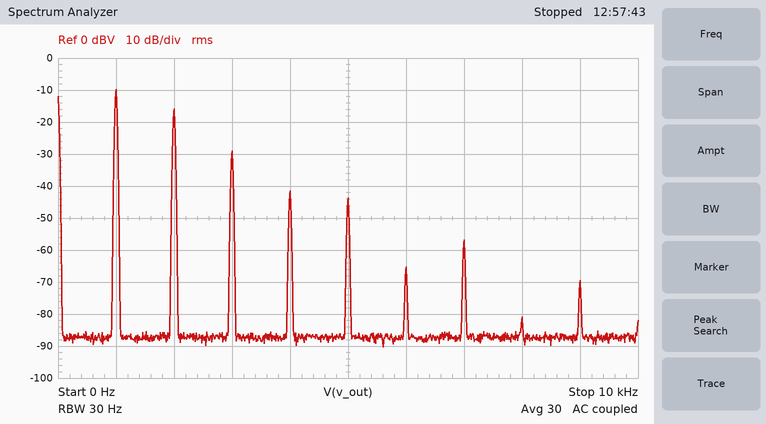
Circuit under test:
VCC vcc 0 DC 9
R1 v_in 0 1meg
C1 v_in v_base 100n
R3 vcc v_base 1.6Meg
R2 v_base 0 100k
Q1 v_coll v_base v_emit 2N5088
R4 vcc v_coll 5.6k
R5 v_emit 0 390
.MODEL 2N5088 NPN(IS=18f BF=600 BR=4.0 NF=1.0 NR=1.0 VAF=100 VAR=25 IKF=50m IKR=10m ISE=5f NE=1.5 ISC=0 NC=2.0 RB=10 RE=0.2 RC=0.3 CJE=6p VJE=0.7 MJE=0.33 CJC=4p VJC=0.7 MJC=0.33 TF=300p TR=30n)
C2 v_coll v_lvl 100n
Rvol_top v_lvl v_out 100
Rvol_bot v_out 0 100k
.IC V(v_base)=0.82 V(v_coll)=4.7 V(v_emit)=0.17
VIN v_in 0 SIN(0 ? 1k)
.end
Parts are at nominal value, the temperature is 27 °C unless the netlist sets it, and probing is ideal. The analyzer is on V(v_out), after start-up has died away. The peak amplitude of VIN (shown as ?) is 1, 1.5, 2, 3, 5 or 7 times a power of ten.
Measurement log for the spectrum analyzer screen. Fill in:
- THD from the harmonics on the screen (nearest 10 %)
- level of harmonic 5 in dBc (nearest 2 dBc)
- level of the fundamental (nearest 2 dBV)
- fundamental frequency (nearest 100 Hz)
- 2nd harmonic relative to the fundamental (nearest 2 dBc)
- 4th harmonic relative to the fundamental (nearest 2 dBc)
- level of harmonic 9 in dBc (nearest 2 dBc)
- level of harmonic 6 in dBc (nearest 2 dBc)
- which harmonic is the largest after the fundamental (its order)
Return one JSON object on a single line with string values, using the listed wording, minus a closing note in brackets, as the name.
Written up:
{"THD from the harmonics on the screen": "50 %", "level of harmonic 5 in dBc": "-34 dBc", "level of the fundamental": "-10 dBV", "fundamental frequency": "1.0 kHz", "2nd harmonic relative to the fundamental": "-6 dBc", "4th harmonic relative to the fundamental": "-32 dBc", "level of harmonic 9 in dBc": "-60 dBc", "level of harmonic 6 in dBc": "-56 dBc", "which harmonic is the largest after the fundamental": "2"}
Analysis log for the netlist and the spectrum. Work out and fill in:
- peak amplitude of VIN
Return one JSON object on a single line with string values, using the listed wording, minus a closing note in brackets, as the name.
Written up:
{"peak amplitude of VIN": "150 mV"}
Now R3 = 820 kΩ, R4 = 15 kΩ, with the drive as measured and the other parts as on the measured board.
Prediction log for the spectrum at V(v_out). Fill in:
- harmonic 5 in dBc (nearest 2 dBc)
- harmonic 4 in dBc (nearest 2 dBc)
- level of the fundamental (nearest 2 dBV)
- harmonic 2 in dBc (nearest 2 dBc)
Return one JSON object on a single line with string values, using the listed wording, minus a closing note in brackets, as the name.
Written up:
{"harmonic 5 in dBc": "-38 dBc", "harmonic 4 in dBc": "-38 dBc", "level of the fundamental": "8 dBV", "harmonic 2 in dBc": "-28 dBc"}
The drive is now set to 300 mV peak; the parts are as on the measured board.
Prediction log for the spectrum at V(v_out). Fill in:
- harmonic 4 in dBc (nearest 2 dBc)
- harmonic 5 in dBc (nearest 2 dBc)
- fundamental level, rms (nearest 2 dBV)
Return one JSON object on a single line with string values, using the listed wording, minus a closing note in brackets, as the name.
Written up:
{"harmonic 4 in dBc": "-26 dBc", "harmonic 5 in dBc": "-28 dBc", "fundamental level, rms": "-2 dBV"}
